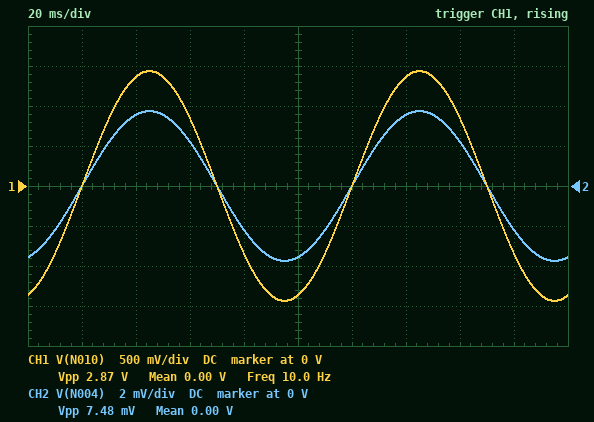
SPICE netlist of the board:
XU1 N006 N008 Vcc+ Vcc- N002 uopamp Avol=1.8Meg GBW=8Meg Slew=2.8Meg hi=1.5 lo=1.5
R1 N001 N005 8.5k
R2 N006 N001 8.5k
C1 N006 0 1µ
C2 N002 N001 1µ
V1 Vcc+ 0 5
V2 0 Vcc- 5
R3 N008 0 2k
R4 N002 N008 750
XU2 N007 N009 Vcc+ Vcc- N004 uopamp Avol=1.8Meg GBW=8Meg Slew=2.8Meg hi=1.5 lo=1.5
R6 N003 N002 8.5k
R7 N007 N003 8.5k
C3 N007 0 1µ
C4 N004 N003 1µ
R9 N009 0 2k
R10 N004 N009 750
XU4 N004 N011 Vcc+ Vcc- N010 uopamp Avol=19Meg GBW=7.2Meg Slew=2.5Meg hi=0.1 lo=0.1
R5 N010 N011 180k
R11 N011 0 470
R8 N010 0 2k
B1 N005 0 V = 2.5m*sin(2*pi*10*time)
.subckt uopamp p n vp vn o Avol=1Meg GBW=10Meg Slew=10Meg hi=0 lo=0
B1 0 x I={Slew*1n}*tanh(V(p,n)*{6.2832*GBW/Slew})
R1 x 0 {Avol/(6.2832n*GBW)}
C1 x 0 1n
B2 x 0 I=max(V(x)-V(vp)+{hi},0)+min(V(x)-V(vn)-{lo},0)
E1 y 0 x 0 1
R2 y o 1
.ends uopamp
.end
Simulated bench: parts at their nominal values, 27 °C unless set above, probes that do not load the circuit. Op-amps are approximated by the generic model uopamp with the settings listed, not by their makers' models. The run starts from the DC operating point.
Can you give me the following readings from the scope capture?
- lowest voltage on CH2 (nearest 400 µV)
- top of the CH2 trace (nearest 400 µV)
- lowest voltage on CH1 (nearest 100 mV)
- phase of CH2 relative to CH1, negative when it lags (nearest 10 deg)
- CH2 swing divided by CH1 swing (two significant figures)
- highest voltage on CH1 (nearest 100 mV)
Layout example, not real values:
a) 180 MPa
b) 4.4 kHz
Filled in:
a) -3.6 mV
b) 3.6 mV
c) -1.4 V
d) 0 deg
e) 0.0026
f) 1.4 V
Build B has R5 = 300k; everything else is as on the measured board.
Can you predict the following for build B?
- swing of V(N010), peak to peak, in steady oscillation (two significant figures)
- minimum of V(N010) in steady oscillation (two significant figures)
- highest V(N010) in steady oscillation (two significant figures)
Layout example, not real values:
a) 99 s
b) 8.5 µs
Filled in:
a) 4.8 V
b) -2.4 V
c) 2.4 V
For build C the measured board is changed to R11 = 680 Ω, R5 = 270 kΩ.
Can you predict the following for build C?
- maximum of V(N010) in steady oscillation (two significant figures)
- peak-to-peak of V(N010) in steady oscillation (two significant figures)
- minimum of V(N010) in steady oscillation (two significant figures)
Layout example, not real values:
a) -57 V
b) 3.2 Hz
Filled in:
a) 1.5 V
b) 3.0 V
c) -1.5 V
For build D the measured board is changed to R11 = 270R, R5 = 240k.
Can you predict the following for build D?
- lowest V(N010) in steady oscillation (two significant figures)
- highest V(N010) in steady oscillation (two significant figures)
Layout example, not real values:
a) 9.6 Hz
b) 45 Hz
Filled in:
a) -3.3 V
b) 3.3 V
